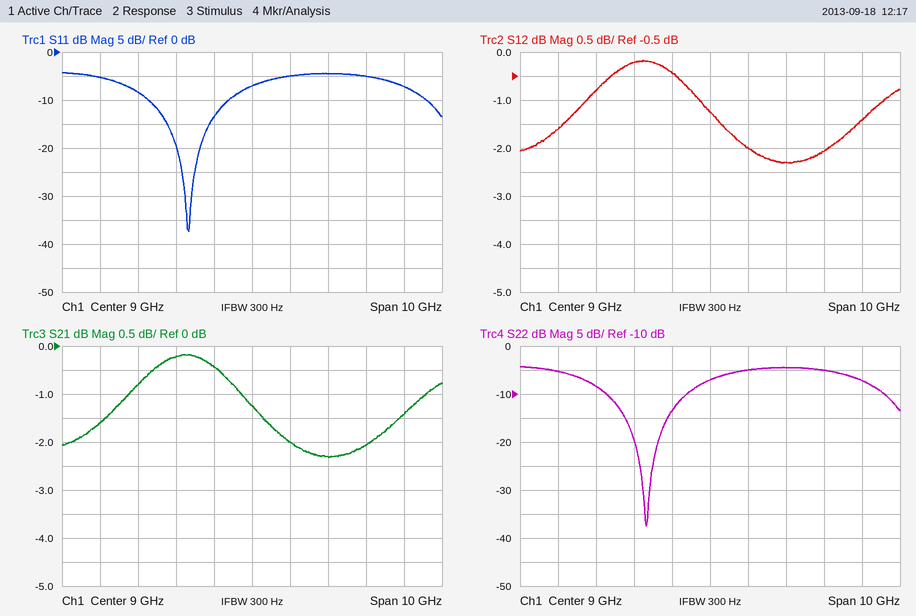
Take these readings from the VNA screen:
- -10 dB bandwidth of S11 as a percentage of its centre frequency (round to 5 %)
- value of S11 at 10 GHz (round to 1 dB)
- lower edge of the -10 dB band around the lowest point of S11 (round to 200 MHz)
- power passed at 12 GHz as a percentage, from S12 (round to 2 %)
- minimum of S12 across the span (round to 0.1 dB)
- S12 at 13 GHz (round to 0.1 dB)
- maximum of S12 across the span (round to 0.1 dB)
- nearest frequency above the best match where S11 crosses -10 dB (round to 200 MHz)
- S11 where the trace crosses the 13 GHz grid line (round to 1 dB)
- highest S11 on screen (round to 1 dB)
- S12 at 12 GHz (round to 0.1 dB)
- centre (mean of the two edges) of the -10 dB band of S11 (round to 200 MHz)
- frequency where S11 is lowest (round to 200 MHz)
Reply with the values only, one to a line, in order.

30 %
-5 dB
6.2 GHz
62 %
-2.3 dB
-1.4 dB
-0.2 dB
8.4 GHz
-7 dB
-4 dB
-2.1 dB
7.4 GHz
7.4 GHz
